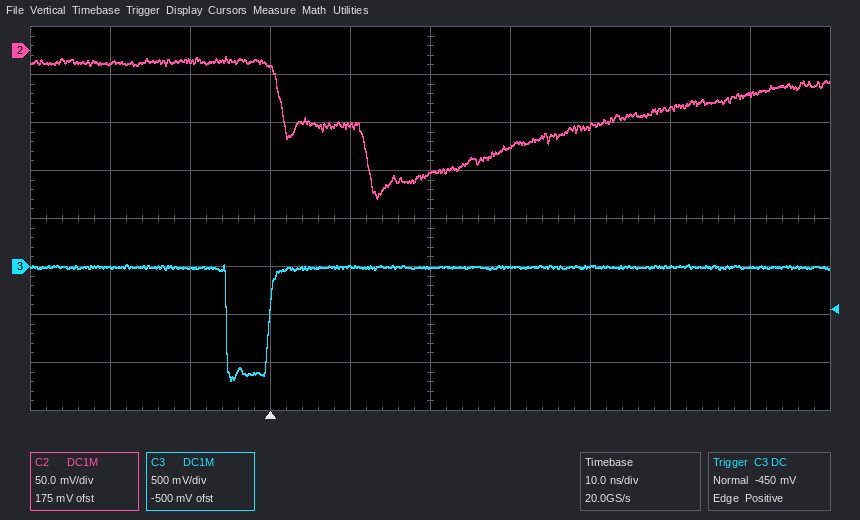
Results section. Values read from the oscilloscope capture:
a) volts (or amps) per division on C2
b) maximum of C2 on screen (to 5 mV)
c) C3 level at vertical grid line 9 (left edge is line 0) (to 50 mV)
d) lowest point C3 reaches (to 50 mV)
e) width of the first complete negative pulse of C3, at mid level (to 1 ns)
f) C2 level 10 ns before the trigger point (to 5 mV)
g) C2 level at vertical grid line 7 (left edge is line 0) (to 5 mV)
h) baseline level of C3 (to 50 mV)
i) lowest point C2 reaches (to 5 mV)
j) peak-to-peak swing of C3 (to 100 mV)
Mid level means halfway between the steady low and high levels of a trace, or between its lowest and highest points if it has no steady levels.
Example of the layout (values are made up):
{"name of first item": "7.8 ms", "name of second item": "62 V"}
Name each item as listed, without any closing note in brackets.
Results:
{"volts (or amps) per division on C2": "50 mV", "maximum of C2 on screen": "-5 mV", "C3 level at vertical grid line 9 (left edge is line 0)": "0 mV", "lowest point C3 reaches": "-1.20 V", "width of the first complete negative pulse of C3, at mid level": "5 ns", "C2 level 10 ns before the trigger point": "-10 mV", "C2 level at vertical grid line 7 (left edge is line 0)": "-80 mV", "baseline level of C3": "0 mV", "lowest point C2 reaches": "-155 mV", "peak-to-peak swing of C3": "1.20 V"}
